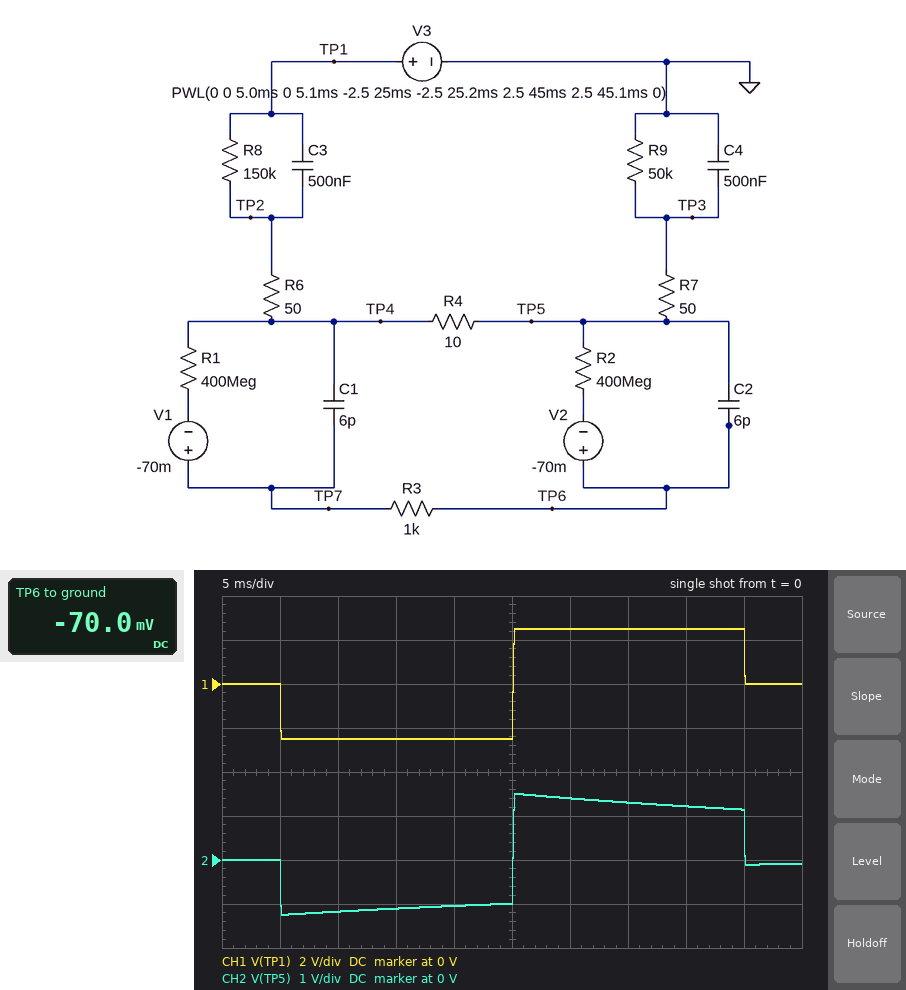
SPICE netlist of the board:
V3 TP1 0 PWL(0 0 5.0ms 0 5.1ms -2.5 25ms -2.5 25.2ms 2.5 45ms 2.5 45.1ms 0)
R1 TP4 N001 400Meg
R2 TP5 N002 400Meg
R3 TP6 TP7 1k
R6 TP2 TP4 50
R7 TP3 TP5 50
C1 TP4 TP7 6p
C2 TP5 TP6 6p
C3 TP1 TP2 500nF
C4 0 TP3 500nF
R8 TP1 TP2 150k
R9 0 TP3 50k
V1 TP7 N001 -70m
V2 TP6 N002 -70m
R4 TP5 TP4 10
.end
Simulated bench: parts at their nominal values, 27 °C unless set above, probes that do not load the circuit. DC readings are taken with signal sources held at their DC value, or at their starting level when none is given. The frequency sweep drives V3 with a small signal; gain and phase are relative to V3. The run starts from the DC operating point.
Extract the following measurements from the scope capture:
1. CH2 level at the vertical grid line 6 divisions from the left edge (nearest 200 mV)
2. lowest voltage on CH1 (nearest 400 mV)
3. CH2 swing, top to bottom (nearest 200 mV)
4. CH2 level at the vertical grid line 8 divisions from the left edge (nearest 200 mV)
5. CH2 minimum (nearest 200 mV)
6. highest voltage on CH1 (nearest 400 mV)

1.4 V
-2.4 V
2.8 V
1.2 V
-1.2 V
2.4 V
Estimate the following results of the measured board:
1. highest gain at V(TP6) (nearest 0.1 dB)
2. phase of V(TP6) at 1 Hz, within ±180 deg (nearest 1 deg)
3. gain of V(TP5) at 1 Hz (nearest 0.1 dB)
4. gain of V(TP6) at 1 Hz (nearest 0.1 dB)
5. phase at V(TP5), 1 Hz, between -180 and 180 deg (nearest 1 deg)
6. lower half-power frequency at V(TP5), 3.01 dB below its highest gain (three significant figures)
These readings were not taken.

-6.0 dB
12 deg
-11.4 dB
-11.4 dB
12 deg
3.00 Hz
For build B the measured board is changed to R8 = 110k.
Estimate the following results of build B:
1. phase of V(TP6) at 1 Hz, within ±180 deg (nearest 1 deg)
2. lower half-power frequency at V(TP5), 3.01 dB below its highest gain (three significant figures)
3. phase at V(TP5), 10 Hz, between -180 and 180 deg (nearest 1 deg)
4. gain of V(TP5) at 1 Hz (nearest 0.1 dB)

7 deg
2.16 Hz
9 deg
-9.8 dB
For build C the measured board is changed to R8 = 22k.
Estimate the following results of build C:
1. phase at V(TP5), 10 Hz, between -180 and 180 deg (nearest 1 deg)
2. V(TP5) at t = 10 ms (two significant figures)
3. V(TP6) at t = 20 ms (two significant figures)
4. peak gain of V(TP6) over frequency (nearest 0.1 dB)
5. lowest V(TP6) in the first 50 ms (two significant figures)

-9 deg
-1.4 V
-1.6 V
-3.2 dB
-1.7 V
